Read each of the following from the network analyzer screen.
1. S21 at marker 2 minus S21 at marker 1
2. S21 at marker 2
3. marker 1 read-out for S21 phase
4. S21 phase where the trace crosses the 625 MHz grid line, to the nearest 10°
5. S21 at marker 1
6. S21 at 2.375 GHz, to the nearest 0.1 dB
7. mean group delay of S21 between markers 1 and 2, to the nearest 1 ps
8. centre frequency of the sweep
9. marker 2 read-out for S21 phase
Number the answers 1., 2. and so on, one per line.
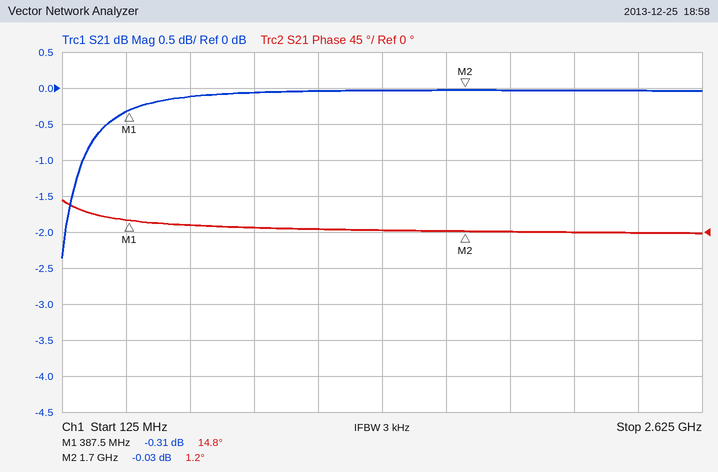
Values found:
1. 0.28 dB
2. -0.03 dB
3. 14.8°
4. 10°
5. -0.31 dB
6. 0.0 dB
7. 29 ps
8. 1.375 GHz
9. 1.2°
